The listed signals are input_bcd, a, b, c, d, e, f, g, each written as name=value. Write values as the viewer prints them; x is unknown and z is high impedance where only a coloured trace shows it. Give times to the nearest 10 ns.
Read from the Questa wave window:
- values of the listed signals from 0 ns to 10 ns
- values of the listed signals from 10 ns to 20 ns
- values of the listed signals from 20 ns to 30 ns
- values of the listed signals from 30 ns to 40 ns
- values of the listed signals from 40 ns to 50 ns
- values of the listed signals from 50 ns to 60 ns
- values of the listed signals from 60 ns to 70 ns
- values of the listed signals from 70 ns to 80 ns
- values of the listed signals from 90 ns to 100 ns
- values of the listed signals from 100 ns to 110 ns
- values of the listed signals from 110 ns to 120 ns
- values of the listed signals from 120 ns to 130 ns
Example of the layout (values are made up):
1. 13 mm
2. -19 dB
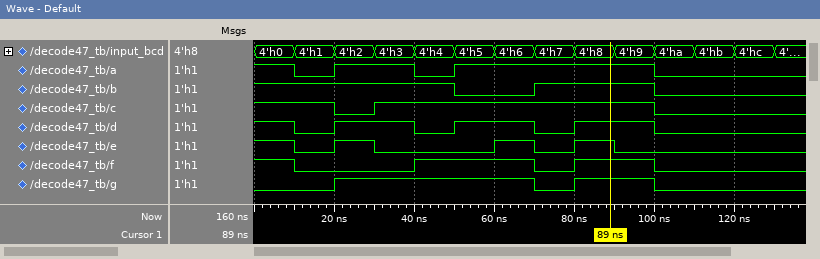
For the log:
1. input_bcd=4'h0, a=1, b=1, c=1, d=1, e=1, f=1, g=0
2. input_bcd=4'h1, a=0, b=1, c=1, d=0, e=0, f=0, g=0
3. input_bcd=4'h2, a=1, b=1, c=0, d=1, e=1, f=0, g=1
4. input_bcd=4'h3, a=1, b=1, c=1, d=1, e=0, f=0, g=1
5. input_bcd=4'h4, a=0, b=1, c=1, d=0, e=0, f=1, g=1
6. input_bcd=4'h5, a=1, b=0, c=1, d=1, e=0, f=1, g=1
7. input_bcd=4'h6, a=1, b=0, c=1, d=1, e=1, f=1, g=1
8. input_bcd=4'h7, a=1, b=1, c=1, d=0, e=0, f=0, g=0
9. input_bcd=4'h9, a=1, b=1, c=1, d=1, e=0, f=1, g=1
10. input_bcd=4'ha, a=0, b=0, c=0, d=0, e=0, f=0, g=0
11. input_bcd=4'hb, a=0, b=0, c=0, d=0, e=0, f=0, g=0
12. input_bcd=4'hc, a=0, b=0, c=0, d=0, e=0, f=0, g=0
